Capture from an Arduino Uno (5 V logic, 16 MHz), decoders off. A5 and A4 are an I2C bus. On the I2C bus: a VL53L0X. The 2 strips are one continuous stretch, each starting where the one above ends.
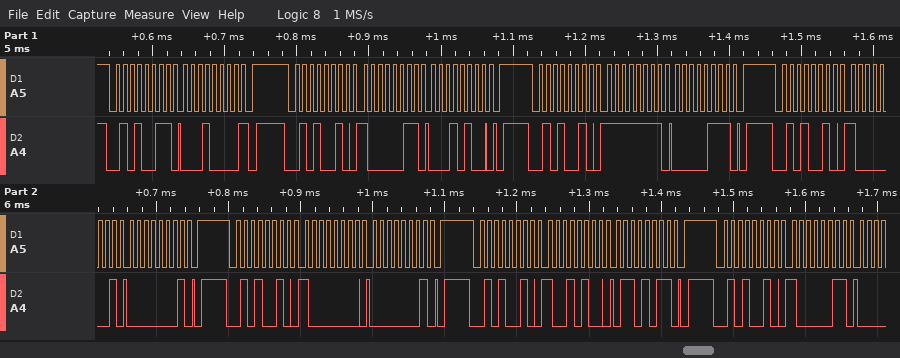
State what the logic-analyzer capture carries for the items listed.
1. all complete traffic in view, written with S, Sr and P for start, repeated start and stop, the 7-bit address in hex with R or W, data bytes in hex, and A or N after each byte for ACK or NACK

S 29R A 10 N P S 29W A 83 A 14 A P S 29W A FF A 07 A P S 29W A 81 A 01 A P S 29W A 80 A 01 A P S 29W A 94 A 6B A P S 29W A 83 A
